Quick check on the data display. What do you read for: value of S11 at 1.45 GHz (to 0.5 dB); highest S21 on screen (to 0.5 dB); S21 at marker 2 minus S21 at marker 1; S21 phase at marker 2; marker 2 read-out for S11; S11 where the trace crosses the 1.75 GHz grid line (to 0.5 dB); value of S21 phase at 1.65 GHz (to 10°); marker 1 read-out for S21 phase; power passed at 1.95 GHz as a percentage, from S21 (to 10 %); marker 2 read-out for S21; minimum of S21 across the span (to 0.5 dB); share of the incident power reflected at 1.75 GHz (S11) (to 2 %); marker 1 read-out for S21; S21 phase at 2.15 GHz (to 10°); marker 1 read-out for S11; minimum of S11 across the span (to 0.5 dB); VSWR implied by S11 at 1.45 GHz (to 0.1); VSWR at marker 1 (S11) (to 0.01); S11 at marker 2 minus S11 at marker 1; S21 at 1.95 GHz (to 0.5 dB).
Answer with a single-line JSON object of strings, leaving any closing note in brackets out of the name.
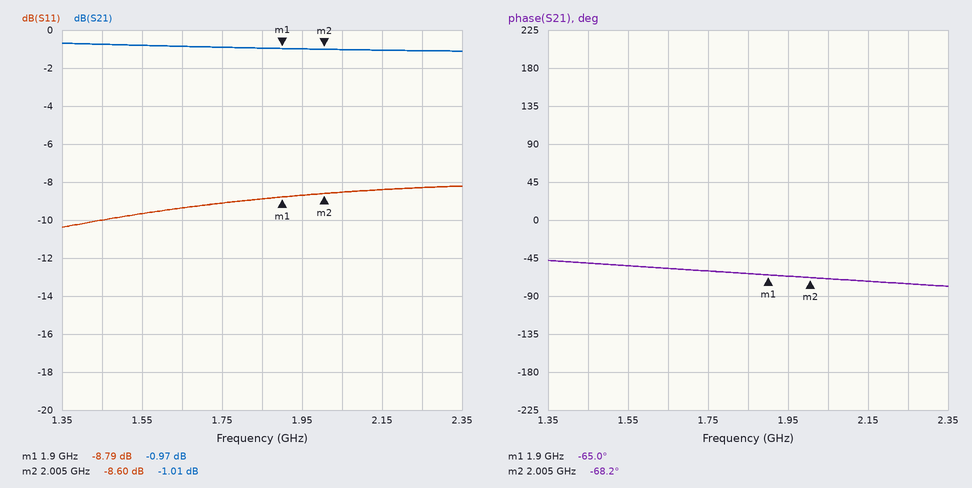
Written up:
{"value of S11 at 1.45 GHz": "-10.0 dB", "highest S21 on screen": "-0.5 dB", "S21 at marker 2 minus S21 at marker 1": "-0.04 dB", "S21 phase at marker 2": "-68.2°", "marker 2 read-out for S11": "-8.60 dB", "S11 where the trace crosses the 1.75 GHz grid line": "-9.0 dB", "value of S21 phase at 1.65 GHz": "-60°", "marker 1 read-out for S21 phase": "-65.0°", "power passed at 1.95 GHz as a percentage, from S21": "80 %", "marker 2 read-out for S21": "-1.01 dB", "minimum of S21 across the span": "-1.0 dB", "share of the incident power reflected at 1.75 GHz (S11)": "12 %", "marker 1 read-out for S21": "-0.97 dB", "S21 phase at 2.15 GHz": "-70°", "marker 1 read-out for S11": "-8.79 dB", "minimum of S11 across the span": "-10.5 dB", "VSWR implied by S11 at 1.45 GHz": "1.9", "VSWR at marker 1 (S11)": "2.14", "S11 at marker 2 minus S11 at marker 1": "0.19 dB", "S21 at 1.95 GHz": "-1.0 dB"}
